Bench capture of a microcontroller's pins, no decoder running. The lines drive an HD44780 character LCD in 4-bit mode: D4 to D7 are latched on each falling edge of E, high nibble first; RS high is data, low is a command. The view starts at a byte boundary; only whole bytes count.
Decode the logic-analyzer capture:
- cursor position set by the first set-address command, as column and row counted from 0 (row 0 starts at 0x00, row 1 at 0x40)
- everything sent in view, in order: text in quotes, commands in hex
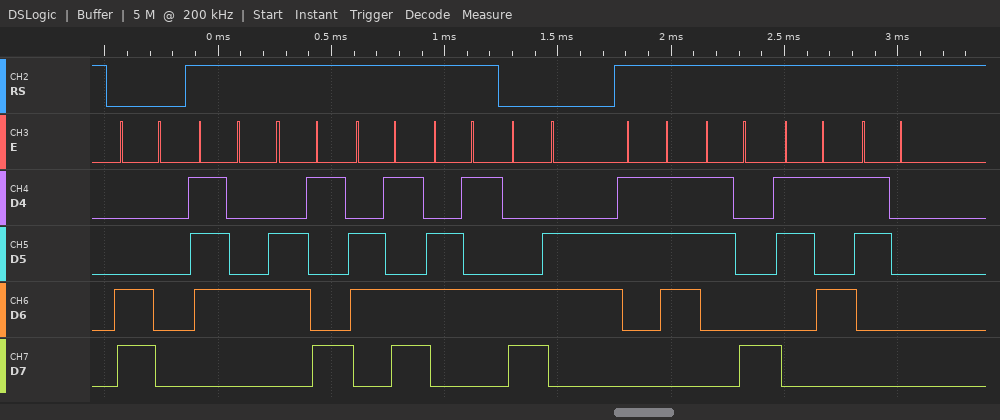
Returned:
column 0, row 1
0xC0 "time" 0xC6 "7850"
